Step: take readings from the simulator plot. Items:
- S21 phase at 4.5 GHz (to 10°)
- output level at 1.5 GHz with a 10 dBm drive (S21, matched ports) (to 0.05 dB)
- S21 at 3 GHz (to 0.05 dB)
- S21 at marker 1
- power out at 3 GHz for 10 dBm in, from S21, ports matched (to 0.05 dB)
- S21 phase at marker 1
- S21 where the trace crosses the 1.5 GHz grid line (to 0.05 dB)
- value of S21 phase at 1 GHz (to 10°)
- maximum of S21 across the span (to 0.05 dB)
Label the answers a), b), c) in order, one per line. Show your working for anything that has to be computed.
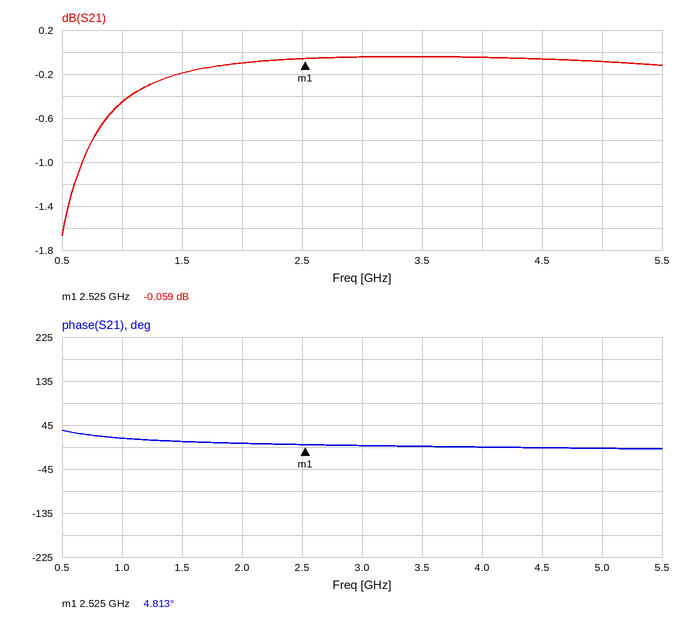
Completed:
a) 0°
b) 10 dBm + (-0.20 dB) = 9.80 dBm
c) -0.05 dB
d) -0.059 dB
e) 10 dBm + (-0.05 dB) = 9.95 dBm
f) 4.813°
g) -0.20 dB
h) 20°
i) -0.05 dB
